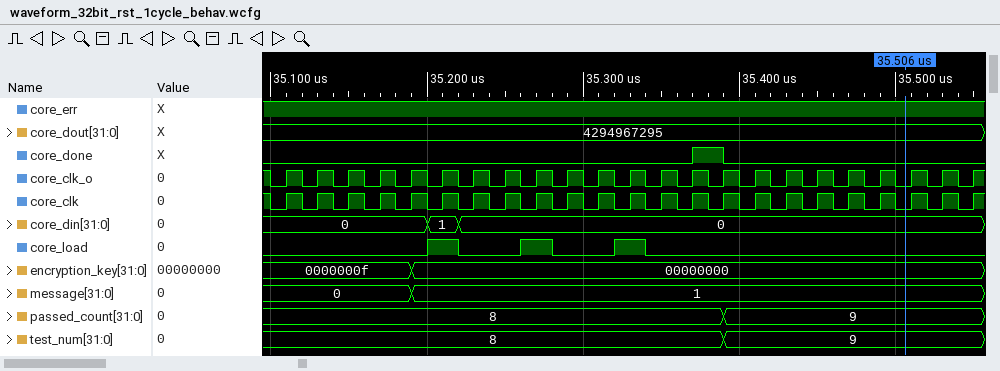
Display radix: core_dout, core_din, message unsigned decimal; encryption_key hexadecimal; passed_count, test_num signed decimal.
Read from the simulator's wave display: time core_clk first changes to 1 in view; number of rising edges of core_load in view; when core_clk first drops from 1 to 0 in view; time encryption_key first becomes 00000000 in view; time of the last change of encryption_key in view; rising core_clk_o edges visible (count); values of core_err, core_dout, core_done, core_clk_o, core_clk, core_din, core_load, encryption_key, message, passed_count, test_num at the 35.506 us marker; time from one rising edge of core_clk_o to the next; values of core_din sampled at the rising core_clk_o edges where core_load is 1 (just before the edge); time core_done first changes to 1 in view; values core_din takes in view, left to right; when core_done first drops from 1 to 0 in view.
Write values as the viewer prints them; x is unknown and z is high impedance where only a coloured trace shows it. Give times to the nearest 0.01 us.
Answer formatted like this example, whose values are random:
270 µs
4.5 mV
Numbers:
35.11 us
3
35.1 us
35.19 us
35.19 us
23
core_err=1, core_dout=4294967295, core_done=0, core_clk_o=0, core_clk=0, core_din=0, core_load=0, encryption_key=00000000, message=1, passed_count=9, test_num=9
0.02 us
1, 0, 0
35.37 us
0, 1, 0
35.39 us
